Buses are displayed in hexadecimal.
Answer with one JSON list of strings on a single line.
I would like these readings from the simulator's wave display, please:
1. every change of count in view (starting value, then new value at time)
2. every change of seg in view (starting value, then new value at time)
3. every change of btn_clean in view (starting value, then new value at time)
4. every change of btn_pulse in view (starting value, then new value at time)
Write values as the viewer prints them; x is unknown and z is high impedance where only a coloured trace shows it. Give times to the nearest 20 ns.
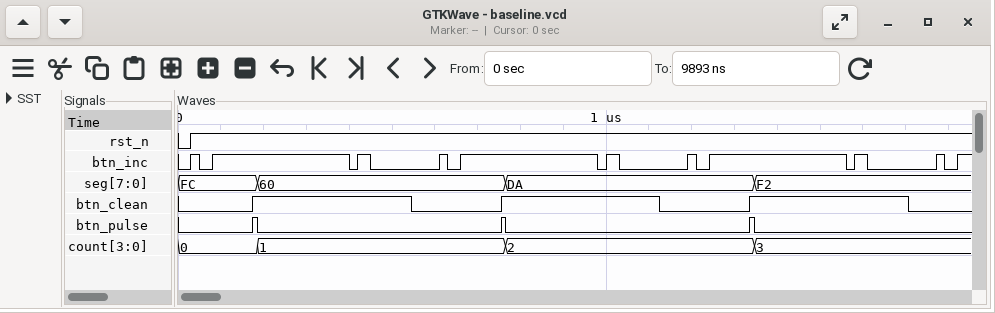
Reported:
["0, 1 at 180 ns, 2 at 760 ns, 3 at 1340 ns", "FC, 60 at 180 ns, DA at 760 ns, F2 at 1340 ns", "0, 1 at 180 ns, 0 at 540 ns, 1 at 760 ns, 0 at 1120 ns, 1 at 1340 ns, 0 at 1700 ns", "0, 1 at 180 ns, 0 at 180 ns, 1 at 760 ns, 0 at 760 ns, 1 at 1340 ns, 0 at 1340 ns"]
